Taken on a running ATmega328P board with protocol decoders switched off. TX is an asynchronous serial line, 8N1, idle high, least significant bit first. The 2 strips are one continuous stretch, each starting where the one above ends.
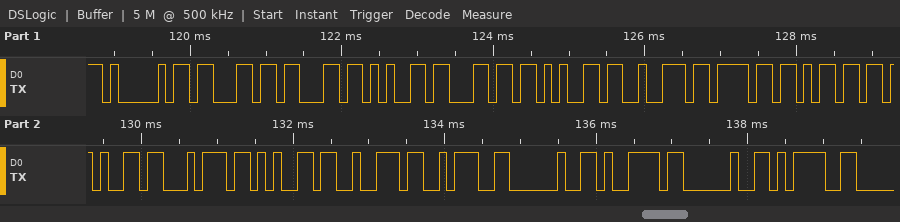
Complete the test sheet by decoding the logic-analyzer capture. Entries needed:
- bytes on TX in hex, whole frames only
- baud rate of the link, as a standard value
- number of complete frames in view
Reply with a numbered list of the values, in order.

1. 0x41 0x63 0x63 0x65 0x6C 0x65 0x72 0x6F 0x6D 0x65 0x74 0x65 0x72 0x3A 0x20 0x79 0x20 0x3D
2. 9600 baud
3. 18
